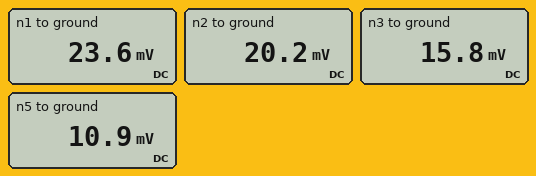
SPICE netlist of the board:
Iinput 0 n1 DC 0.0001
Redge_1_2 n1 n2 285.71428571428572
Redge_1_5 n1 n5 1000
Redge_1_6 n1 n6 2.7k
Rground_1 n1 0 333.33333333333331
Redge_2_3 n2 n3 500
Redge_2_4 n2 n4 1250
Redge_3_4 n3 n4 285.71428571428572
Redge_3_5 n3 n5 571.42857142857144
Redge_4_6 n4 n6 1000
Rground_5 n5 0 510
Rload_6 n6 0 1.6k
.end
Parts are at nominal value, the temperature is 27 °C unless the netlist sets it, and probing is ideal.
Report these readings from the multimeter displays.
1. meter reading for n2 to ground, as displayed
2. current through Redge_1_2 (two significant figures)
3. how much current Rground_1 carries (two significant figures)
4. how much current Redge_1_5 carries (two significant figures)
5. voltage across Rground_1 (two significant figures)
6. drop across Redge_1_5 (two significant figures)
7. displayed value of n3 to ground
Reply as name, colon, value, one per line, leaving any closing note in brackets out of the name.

meter reading for n2 to ground, as displayed: 20.2 mV
current through Redge_1_2: 12 µA
how much current Rground_1 carries: 71 µA
how much current Redge_1_5 carries: 13 µA
voltage across Rground_1: 24 mV
drop across Redge_1_5: 13 mV
displayed value of n3 to ground: 15.8 mV
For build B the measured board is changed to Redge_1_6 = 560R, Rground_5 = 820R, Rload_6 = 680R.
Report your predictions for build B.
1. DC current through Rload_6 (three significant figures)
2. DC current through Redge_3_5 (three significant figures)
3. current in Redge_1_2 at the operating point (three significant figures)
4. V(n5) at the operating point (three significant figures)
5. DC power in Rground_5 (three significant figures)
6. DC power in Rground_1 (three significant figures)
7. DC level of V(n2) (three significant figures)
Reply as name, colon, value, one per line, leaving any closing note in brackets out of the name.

DC current through Rload_6: 19.0 µA
DC current through Redge_3_5: 6.07 µA
current in Redge_1_2 at the operating point: 9.10 µA
V(n5) at the operating point: 12.6 mV
DC power in Rground_5: 193 nW
DC power in Rground_1: 1.44 µW
DC level of V(n2): 19.3 mV
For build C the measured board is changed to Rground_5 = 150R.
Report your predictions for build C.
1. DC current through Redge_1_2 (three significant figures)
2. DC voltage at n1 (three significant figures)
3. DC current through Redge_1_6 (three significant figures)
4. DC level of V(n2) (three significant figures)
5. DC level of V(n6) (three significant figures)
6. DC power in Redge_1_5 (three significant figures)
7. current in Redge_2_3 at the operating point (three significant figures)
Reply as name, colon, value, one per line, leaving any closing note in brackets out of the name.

DC current through Redge_1_2: 14.8 µA
DC voltage at n1: 21.4 mV
DC current through Redge_1_6: 4.18 µA
DC level of V(n2): 17.1 mV
DC level of V(n6): 10.1 mV
DC power in Redge_1_5: 286 nW
current in Redge_2_3 at the operating point: 10.9 µA
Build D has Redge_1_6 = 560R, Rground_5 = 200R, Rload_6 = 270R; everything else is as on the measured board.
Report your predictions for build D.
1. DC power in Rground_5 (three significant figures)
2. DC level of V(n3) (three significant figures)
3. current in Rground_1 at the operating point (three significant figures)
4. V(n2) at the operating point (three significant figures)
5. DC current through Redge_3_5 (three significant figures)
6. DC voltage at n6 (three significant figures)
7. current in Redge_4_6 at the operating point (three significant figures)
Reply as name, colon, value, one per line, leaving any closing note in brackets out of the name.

DC power in Rground_5: 102 nW
DC level of V(n3): 9.77 mV
current in Rground_1 at the operating point: 53.6 µA
V(n2) at the operating point: 14.3 mV
DC current through Redge_3_5: 9.20 µA
DC voltage at n6: 6.43 mV
current in Redge_4_6 at the operating point: 3.39 µA
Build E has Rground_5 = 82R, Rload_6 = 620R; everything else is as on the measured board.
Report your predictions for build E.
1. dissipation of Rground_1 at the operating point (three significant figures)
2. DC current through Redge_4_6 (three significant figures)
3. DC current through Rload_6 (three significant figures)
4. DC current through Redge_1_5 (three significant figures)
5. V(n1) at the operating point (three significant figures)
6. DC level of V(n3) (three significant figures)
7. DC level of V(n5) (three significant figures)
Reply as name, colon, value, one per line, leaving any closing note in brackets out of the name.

dissipation of Rground_1 at the operating point: 1.22 µW
DC current through Redge_4_6: 3.98 µA
DC current through Rload_6: 9.31 µA
DC current through Redge_1_5: 17.7 µA
V(n1) at the operating point: 20.2 mV
DC level of V(n3): 9.58 mV
DC level of V(n5): 2.47 mV
